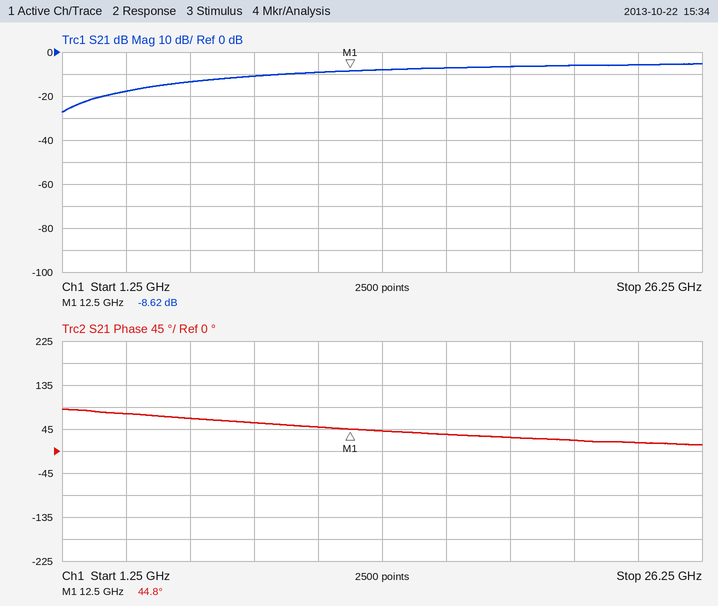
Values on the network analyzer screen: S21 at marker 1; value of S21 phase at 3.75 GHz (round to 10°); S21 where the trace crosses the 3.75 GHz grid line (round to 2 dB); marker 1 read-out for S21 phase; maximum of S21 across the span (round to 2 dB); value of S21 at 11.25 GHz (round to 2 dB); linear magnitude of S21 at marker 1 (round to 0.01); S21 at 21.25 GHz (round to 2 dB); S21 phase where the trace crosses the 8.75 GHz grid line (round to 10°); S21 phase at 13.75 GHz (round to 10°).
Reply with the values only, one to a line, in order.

-8.62 dB
80°
-18 dB
44.8°
-6 dB
-10 dB
0.37
-6 dB
60°
40°
